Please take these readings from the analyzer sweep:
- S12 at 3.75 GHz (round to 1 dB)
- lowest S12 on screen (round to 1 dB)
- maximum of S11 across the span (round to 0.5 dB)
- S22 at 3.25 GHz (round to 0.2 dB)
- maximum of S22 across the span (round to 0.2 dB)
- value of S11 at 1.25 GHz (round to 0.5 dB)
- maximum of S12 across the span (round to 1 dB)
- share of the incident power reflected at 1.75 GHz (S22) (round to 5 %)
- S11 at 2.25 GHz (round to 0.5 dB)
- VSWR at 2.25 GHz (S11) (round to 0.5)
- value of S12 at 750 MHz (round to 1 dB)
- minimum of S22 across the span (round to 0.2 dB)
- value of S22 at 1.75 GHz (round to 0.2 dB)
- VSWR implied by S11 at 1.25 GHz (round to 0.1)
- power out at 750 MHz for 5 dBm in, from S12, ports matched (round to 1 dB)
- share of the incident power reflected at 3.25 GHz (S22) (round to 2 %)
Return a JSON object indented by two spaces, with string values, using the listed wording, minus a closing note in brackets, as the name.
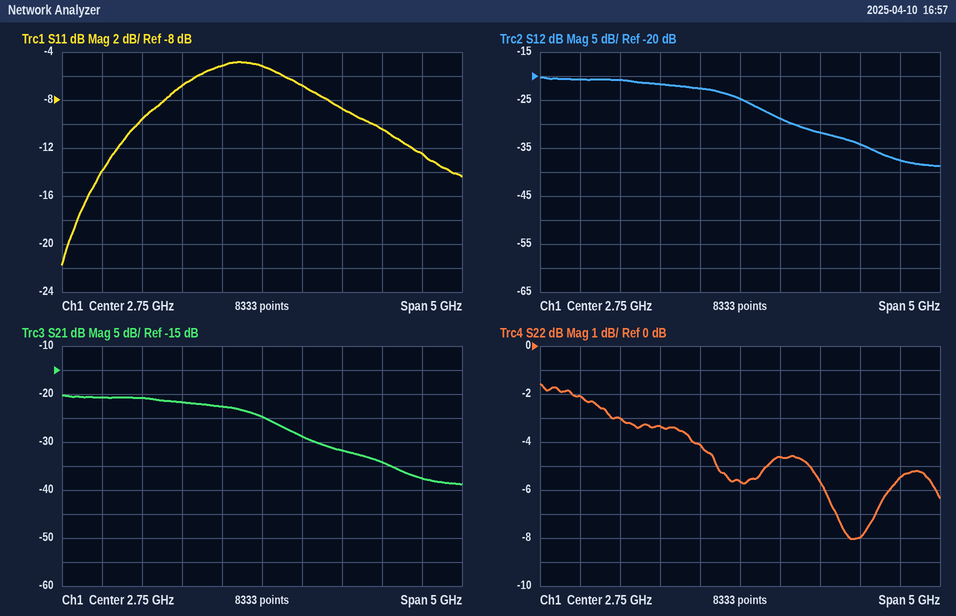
{
  "S12 at 3.75 GHz": "-32 dB",
  "lowest S12 on screen": "-39 dB",
  "maximum of S11 across the span": "-5.0 dB",
  "S22 at 3.25 GHz": "-4.6 dB",
  "maximum of S22 across the span": "-1.6 dB",
  "value of S11 at 1.25 GHz": "-9.5 dB",
  "maximum of S12 across the span": "-20 dB",
  "share of the incident power reflected at 1.75 GHz (S22)": "45 %",
  "S11 at 2.25 GHz": "-5.0 dB",
  "VSWR at 2.25 GHz (S11)": "3.5",
  "value of S12 at 750 MHz": "-21 dB",
  "minimum of S22 across the span": "-8.0 dB",
  "value of S22 at 1.75 GHz": "-3.4 dB",
  "VSWR implied by S11 at 1.25 GHz": "2.0",
  "power out at 750 MHz for 5 dBm in, from S12, ports matched": "-16 dBm",
  "share of the incident power reflected at 3.25 GHz (S22)": "34 %"
}
